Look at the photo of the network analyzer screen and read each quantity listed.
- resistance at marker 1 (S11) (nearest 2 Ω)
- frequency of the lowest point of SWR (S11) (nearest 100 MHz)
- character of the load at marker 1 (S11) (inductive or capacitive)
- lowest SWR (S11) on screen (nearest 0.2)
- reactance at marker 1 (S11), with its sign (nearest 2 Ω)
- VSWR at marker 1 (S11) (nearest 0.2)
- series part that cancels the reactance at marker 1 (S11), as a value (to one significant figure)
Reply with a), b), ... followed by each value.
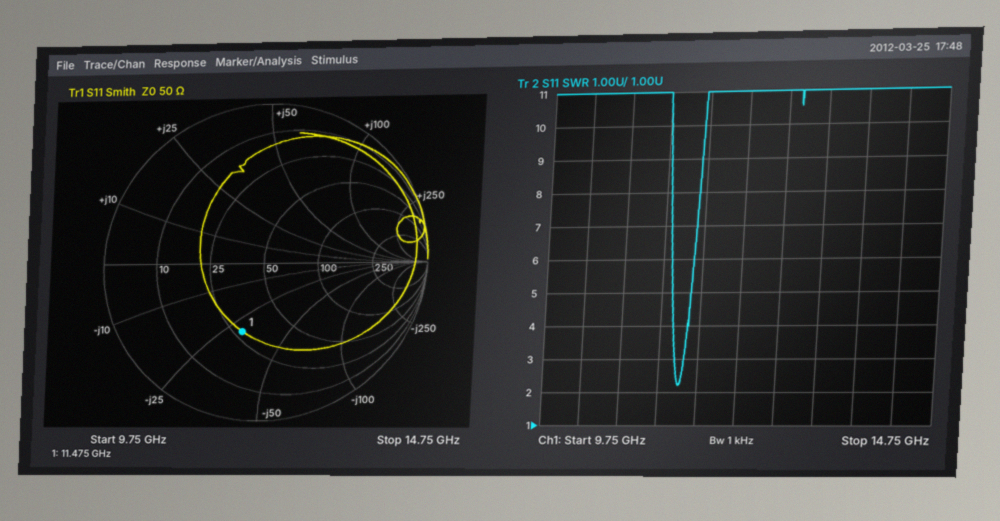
a) 28 Ω
b) 11.5 GHz
c) capacitive
d) 2.2
e) -30 Ω
f) 2.6
g) 400 pH
